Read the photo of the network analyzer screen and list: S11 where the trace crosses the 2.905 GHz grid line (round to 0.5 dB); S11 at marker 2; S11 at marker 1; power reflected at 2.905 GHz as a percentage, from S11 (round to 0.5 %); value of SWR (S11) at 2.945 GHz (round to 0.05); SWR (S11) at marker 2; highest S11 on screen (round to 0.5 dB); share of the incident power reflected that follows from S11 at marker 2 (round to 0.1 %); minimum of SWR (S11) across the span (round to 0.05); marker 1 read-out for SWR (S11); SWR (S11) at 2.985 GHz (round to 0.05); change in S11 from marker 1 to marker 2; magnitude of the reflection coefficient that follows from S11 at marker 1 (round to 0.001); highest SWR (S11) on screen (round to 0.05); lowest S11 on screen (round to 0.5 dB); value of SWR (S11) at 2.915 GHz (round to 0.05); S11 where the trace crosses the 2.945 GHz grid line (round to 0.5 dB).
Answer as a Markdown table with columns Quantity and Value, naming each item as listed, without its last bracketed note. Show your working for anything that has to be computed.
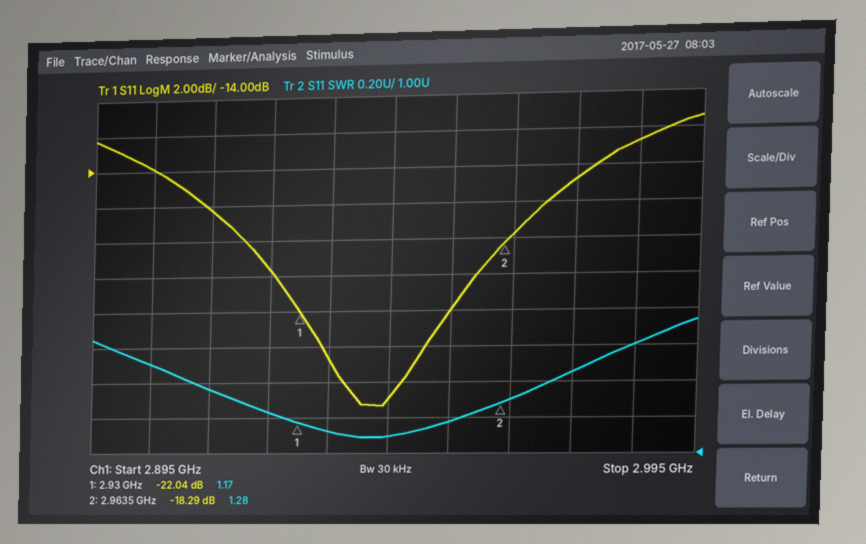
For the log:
| Quantity | Value |
|---|---|
| S11 where the trace crosses the 2.905 GHz grid line | -14.0 dB |
| S11 at marker 2 | -18.29 dB |
| S11 at marker 1 | -22.04 dB |
| power reflected at 2.905 GHz as a percentage, from S11 | 10^(-14/10) ≈ 4.0 % |
| value of SWR (S11) at 2.945 GHz | 1.10 |
| SWR (S11) at marker 2 | 1.28 |
| highest S11 on screen | -11.5 dB |
| share of the incident power reflected that follows from S11 at marker 2 | 10^(-18.29/10) ≈ 1.5 % |
| minimum of SWR (S11) across the span | 1.10 |
| marker 1 read-out for SWR | 1.17 |
| SWR (S11) at 2.985 GHz | 1.60 |
| change in S11 from marker 1 to marker 2 | -18.29 − (-22.04) = 3.75 dB |
| magnitude of the reflection coefficient that follows from S11 at marker 1 | 10^(-22.04/20) ≈ 0.079 |
| highest SWR (S11) on screen | 1.75 |
| lowest S11 on screen | -27.5 dB |
| value of SWR (S11) at 2.915 GHz | 1.35 |
| S11 where the trace crosses the 2.945 GHz grid line | -27.0 dB |
